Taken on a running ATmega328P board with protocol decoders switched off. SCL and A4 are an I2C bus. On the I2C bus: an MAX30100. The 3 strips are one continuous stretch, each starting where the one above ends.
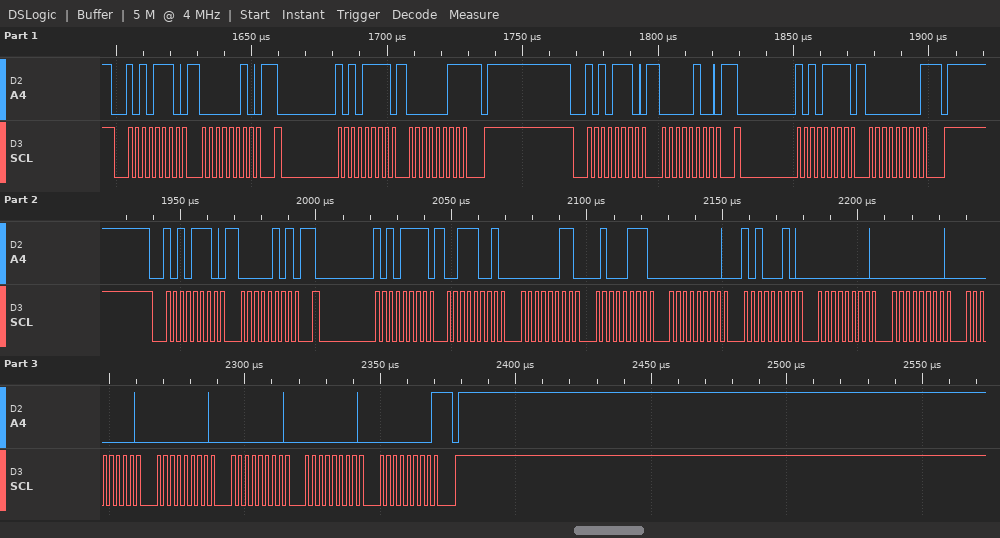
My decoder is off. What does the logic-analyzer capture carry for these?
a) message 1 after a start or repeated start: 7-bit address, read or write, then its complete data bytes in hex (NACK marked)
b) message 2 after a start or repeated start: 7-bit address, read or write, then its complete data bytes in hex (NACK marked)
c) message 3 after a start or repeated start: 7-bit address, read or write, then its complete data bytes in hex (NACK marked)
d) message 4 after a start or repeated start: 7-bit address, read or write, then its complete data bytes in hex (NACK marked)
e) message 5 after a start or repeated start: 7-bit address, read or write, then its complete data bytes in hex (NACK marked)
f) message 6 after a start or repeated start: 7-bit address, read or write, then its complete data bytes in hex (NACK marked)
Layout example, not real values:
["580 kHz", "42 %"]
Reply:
["0x57 write: 02", "0x57 read: 03 NACK", "0x57 write: 04", "0x57 read: 00 NACK", "0x57 write: 05", "0x57 read: 39 03 47 00 A2 00 00 00 00 00 00 00 NACK"]
